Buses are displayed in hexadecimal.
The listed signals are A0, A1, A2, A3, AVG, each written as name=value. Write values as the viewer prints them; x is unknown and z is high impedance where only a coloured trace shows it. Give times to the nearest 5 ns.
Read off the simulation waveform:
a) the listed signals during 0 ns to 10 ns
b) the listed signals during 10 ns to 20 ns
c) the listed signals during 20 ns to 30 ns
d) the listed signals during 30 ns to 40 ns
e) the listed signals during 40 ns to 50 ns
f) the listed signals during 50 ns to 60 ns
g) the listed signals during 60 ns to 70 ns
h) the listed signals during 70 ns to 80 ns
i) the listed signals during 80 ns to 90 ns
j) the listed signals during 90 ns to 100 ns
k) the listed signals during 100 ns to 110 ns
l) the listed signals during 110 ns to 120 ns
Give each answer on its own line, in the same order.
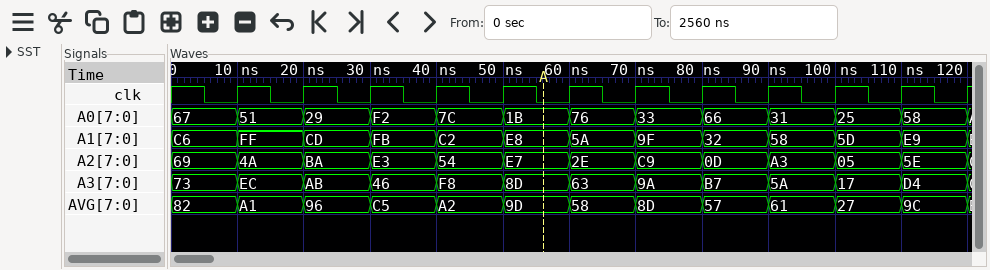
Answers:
A0=67, A1=C6, A2=69, A3=73, AVG=82
A0=51, A1=FF, A2=4A, A3=EC, AVG=A1
A0=29, A1=CD, A2=BA, A3=AB, AVG=96
A0=F2, A1=FB, A2=E3, A3=46, AVG=C5
A0=7C, A1=C2, A2=54, A3=F8, AVG=A2
A0=1B, A1=E8, A2=E7, A3=8D, AVG=9D
A0=76, A1=5A, A2=2E, A3=63, AVG=58
A0=33, A1=9F, A2=C9, A3=9A, AVG=8D
A0=66, A1=32, A2=0D, A3=B7, AVG=57
A0=31, A1=58, A2=A3, A3=5A, AVG=61
A0=25, A1=5D, A2=05, A3=17, AVG=27
A0=58, A1=E9, A2=5E, A3=D4, AVG=9C
